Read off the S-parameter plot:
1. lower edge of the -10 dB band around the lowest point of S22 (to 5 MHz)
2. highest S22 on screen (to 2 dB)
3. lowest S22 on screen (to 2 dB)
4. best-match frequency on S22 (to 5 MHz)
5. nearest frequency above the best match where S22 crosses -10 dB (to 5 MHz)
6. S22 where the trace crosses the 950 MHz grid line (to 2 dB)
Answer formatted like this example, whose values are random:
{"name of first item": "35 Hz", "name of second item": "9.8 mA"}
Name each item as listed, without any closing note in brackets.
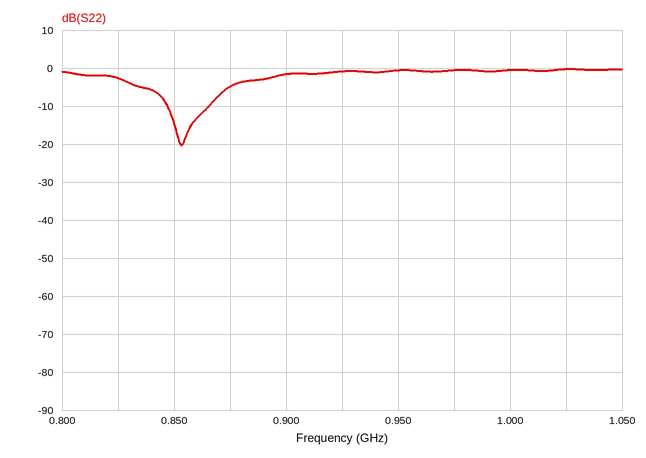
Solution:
{"lower edge of the -10 dB band around the lowest point of S22": "845 MHz", "highest S22 on screen": "0 dB", "lowest S22 on screen": "-20 dB", "best-match frequency on S22": "855 MHz", "nearest frequency above the best match where S22 crosses -10 dB": "865 MHz", "S22 where the trace crosses the 950 MHz grid line": "0 dB"}
